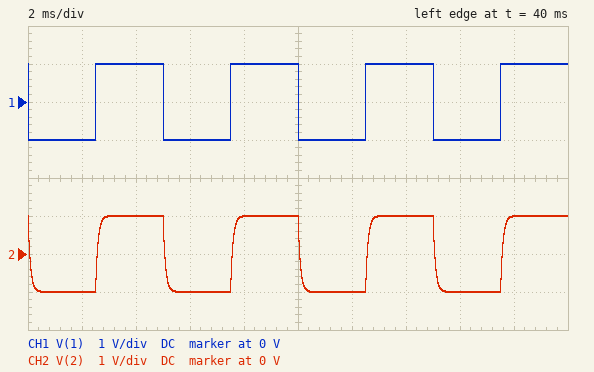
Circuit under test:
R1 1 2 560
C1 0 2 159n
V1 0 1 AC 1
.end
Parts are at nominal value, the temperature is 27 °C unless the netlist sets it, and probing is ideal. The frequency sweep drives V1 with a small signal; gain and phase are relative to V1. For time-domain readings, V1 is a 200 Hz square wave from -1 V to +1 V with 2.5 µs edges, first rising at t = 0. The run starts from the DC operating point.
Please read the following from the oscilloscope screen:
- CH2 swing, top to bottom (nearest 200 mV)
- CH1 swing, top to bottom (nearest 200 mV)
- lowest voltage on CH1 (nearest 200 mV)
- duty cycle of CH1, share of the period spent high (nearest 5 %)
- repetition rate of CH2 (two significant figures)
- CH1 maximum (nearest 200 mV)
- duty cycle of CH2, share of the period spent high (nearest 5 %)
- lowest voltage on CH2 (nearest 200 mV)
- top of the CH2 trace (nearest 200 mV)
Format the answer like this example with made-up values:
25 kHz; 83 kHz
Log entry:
2.0 V; 2.0 V; -1.0 V; 50 %; 200 Hz; 1.0 V; 50 %; -1.0 V; 1.0 V
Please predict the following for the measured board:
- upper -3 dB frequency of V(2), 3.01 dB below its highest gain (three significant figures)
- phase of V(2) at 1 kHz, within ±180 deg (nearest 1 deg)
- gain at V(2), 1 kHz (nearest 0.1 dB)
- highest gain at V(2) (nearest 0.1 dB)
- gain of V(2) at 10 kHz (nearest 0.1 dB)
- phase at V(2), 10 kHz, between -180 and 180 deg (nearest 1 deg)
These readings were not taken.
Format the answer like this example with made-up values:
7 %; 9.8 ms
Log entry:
1.79 kHz; 151 deg; -1.2 dB; 0 dB; -15.1 dB; 100 deg
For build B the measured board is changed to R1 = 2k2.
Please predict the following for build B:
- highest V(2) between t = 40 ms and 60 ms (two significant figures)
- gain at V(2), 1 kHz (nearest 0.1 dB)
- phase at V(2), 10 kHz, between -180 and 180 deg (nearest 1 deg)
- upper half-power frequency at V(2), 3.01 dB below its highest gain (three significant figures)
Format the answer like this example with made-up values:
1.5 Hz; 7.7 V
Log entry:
1.0 V; -7.7 dB; 93 deg; 455 Hz
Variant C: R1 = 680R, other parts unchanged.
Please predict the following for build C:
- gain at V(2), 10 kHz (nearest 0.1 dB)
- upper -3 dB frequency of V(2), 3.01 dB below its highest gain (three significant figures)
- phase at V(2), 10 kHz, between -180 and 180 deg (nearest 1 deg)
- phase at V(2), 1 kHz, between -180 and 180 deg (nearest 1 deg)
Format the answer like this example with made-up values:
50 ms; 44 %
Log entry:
-16.7 dB; 1.47 kHz; 98 deg; 146 deg
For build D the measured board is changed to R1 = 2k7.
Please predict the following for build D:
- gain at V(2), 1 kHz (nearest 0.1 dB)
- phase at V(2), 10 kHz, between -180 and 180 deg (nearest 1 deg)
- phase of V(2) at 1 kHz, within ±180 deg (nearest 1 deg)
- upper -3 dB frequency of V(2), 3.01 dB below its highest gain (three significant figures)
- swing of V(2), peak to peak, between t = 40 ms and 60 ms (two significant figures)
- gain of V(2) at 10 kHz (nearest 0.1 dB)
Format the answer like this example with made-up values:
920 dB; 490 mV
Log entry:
-9.2 dB; 92 deg; 110 deg; 371 Hz; 2.0 V; -28.6 dB
